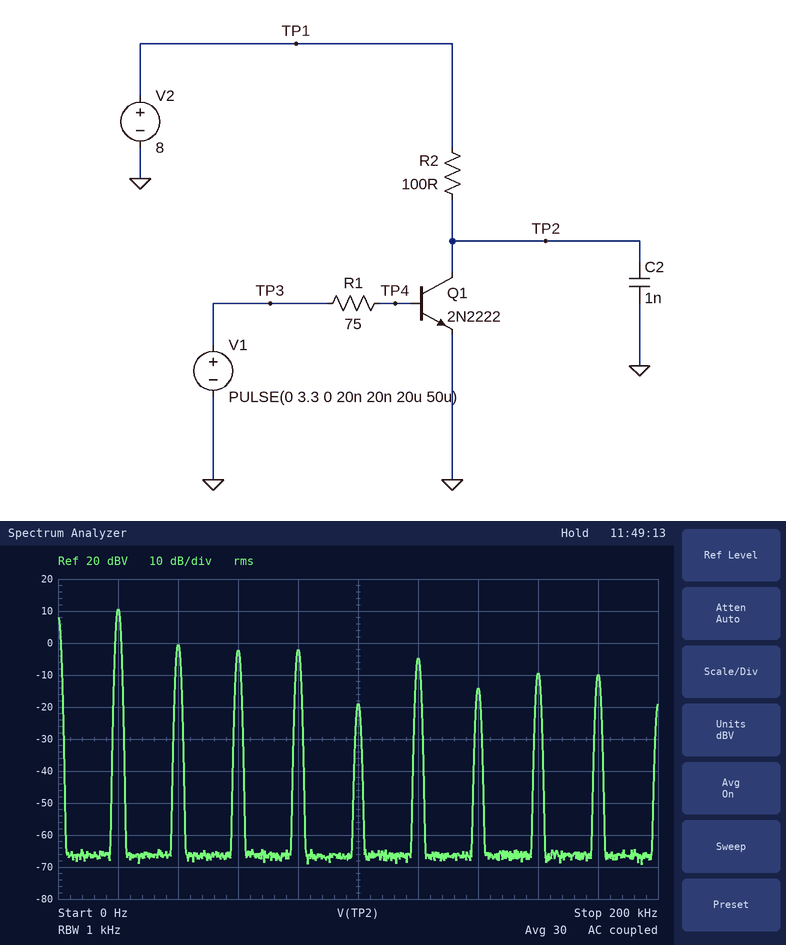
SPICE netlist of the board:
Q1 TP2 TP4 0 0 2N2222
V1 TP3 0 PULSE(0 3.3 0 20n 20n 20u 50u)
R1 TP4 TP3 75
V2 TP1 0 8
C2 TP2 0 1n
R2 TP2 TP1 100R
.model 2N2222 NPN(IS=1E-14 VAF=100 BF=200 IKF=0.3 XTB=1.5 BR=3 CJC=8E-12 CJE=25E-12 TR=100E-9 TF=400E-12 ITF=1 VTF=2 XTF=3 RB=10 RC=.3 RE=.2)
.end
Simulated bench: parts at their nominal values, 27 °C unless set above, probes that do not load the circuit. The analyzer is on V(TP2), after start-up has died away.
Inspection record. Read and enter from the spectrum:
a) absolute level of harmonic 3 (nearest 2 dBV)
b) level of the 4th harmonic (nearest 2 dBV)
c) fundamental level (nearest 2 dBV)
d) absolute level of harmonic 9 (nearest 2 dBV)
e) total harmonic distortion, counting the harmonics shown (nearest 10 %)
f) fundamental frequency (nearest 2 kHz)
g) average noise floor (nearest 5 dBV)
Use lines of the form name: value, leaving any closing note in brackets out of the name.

absolute level of harmonic 3: -2 dBV
level of the 4th harmonic: -2 dBV
fundamental level: 10 dBV
absolute level of harmonic 9: -10 dBV
total harmonic distortion, counting the harmonics shown: 50 %
fundamental frequency: 20 kHz
average noise floor: -65 dBV
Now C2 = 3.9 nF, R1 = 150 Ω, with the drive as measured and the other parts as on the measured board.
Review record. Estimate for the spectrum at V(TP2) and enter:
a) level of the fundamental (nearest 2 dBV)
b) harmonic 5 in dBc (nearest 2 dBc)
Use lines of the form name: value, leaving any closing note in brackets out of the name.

level of the fundamental: 10 dBV
harmonic 5 in dBc: -26 dBc
